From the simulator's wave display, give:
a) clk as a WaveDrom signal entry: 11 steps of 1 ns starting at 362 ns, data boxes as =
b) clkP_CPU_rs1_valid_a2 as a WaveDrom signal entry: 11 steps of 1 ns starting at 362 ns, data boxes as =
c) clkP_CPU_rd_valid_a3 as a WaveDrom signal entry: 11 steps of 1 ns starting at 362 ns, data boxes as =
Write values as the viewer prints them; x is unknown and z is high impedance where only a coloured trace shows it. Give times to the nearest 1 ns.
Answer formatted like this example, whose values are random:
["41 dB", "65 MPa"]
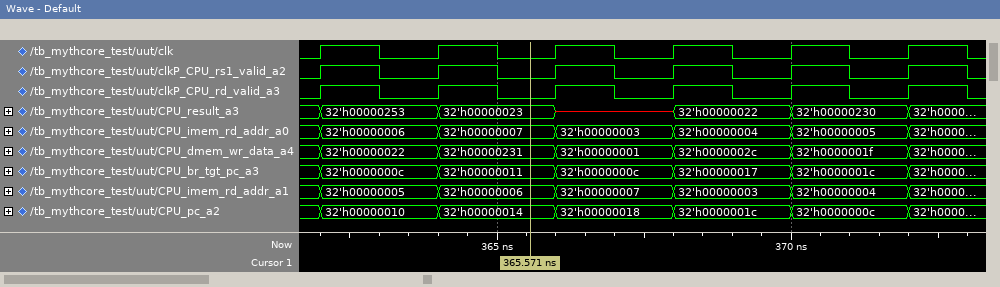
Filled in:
["{name: 'clk', wave: '10101010101'}", "{name: 'clkP_CPU_rs1_valid_a2', wave: '10101010101'}", "{name: 'clkP_CPU_rd_valid_a3', wave: '10101010101'}"]
